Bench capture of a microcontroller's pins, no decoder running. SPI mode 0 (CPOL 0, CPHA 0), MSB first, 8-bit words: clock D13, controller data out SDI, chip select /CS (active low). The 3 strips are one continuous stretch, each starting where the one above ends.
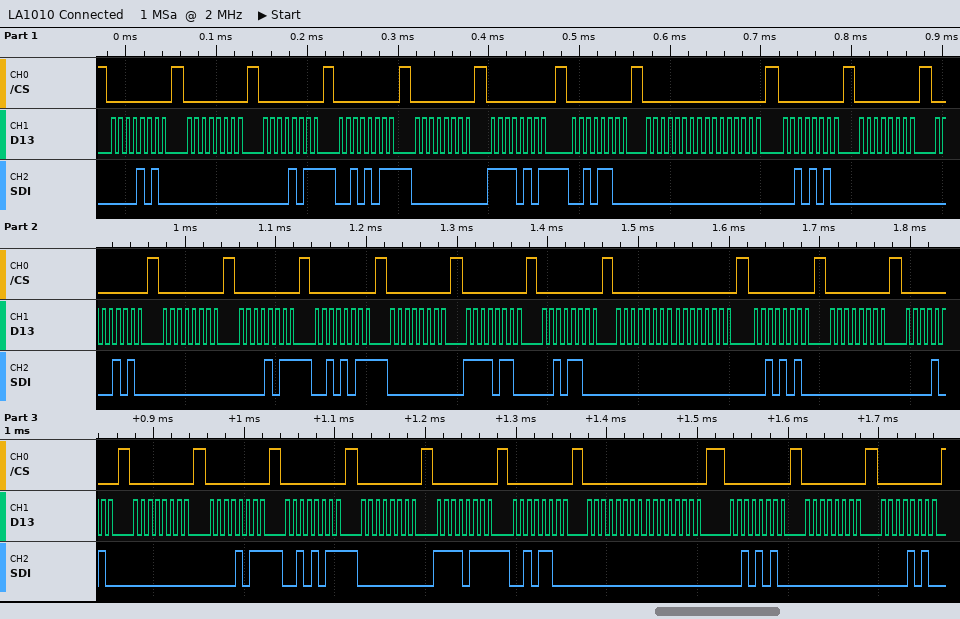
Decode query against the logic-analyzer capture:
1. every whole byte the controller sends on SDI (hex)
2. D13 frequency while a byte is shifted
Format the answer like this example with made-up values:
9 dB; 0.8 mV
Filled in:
0A 00 0B 2B 00 F5 2C 00 00 2A 00 0A 00 0B 2B 00 F6 2C 00 00 2A 00 0A 00 0B 2B 00 F7 2C 00 00 2A 00 0A; 125 kHz
